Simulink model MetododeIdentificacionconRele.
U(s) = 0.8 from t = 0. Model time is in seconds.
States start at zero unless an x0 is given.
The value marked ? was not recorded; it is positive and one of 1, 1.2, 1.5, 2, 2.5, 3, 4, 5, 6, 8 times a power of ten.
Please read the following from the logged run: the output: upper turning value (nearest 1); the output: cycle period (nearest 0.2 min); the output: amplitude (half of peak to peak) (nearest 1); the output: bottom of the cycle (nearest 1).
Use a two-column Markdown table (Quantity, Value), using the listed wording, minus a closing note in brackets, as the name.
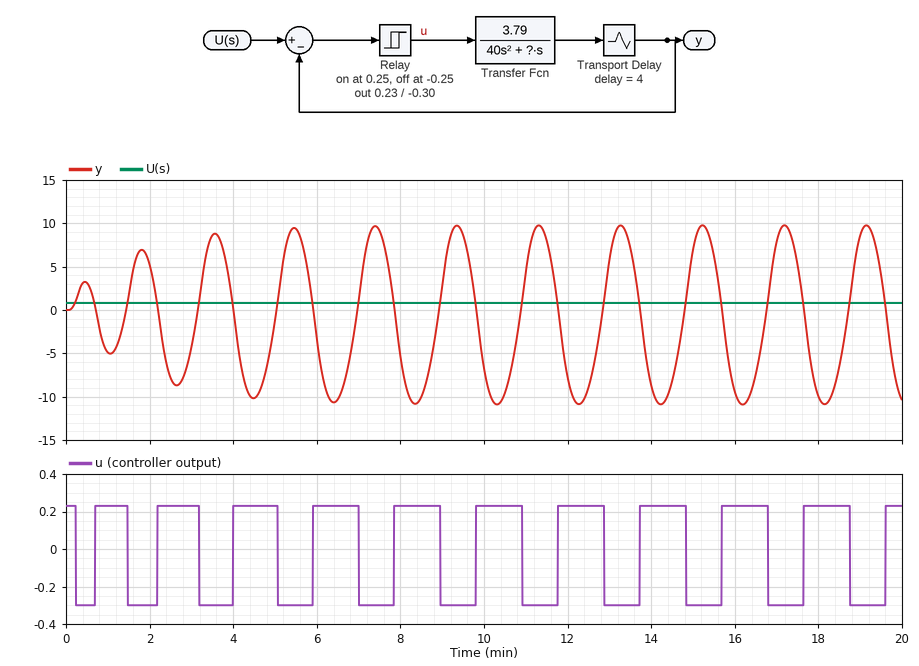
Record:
| Quantity | Value |
|---|---|
| the output: upper turning value | 10 |
| the output: cycle period | 2.0 min |
| the output: amplitude (half of peak to peak) | 10 |
| the output: bottom of the cycle | -11 |
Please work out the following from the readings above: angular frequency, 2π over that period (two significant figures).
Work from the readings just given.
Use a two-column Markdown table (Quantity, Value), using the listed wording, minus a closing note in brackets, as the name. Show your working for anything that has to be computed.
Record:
| Quantity | Value |
|---|---|
| angular frequency, 2π over that period | 2π / 2 = 3.1 rad/min |
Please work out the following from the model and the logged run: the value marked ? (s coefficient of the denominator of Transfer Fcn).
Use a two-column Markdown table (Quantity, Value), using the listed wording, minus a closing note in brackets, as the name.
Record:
| Quantity | Value |
|---|---|
| the value marked ? | 0.6 |
